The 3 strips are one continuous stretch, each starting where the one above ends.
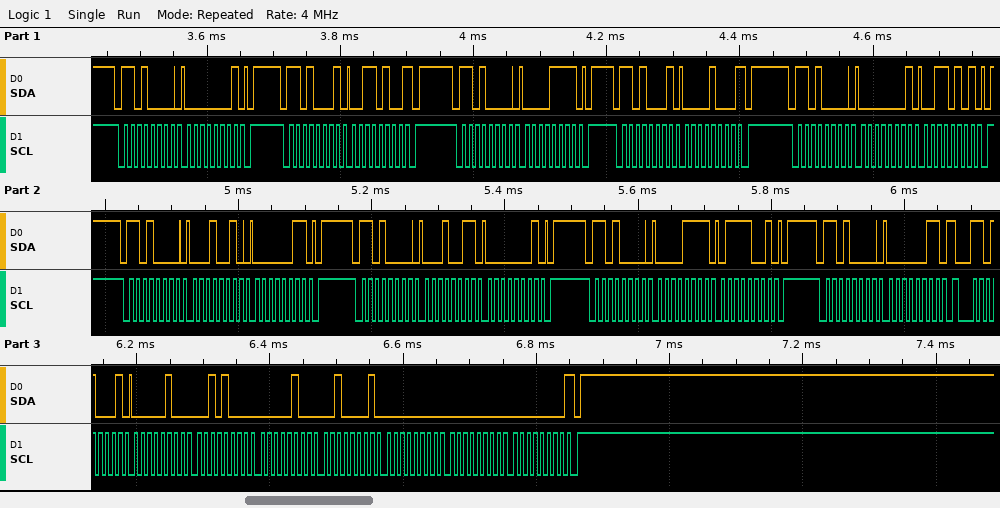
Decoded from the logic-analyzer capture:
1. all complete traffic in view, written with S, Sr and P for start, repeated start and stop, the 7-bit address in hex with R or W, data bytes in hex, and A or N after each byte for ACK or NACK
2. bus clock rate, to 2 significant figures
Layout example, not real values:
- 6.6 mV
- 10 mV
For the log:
- S 68W A 01 A P S 68R A 34 N P S 68W A 0F A P S 68R A 08 N P S 68W A 01 A 35 A P S 68W A 12 A 03 A P S 68W A 13 A 01 A P S 68W A 0F A 79 A P S 68W A 03 A Sr 68R A 04 A 28 A 04 A 21 A 00 A 00 A 00 N P
- 100 kHz
